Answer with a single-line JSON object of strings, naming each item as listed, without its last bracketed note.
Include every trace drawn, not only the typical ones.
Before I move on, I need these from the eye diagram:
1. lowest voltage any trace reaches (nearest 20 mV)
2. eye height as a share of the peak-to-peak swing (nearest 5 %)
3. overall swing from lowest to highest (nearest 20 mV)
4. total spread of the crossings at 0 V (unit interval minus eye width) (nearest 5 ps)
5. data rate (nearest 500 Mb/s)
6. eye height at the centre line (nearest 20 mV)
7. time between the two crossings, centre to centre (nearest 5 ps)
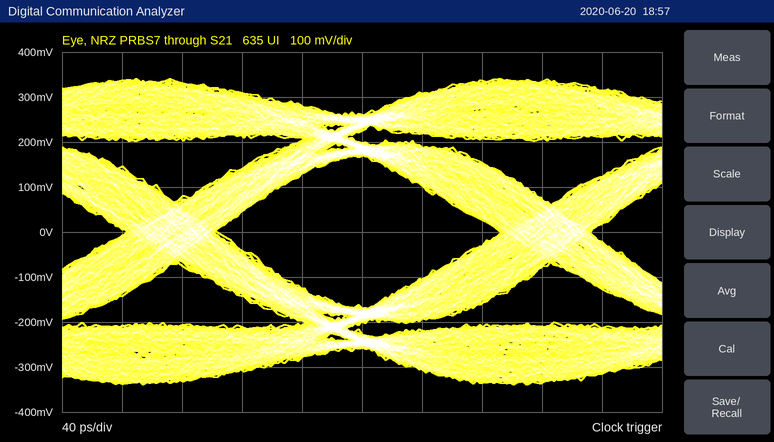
{"lowest voltage any trace reaches": "-340 mV", "eye height as a share of the peak-to-peak swing": "50 %", "overall swing from lowest to highest": "680 mV", "total spread of the crossings at 0 V (unit interval minus eye width)": "60 ps", "data rate": "4.0 Gb/s", "eye height at the centre line": "340 mV", "time between the two crossings, centre to centre": "250 ps"}
